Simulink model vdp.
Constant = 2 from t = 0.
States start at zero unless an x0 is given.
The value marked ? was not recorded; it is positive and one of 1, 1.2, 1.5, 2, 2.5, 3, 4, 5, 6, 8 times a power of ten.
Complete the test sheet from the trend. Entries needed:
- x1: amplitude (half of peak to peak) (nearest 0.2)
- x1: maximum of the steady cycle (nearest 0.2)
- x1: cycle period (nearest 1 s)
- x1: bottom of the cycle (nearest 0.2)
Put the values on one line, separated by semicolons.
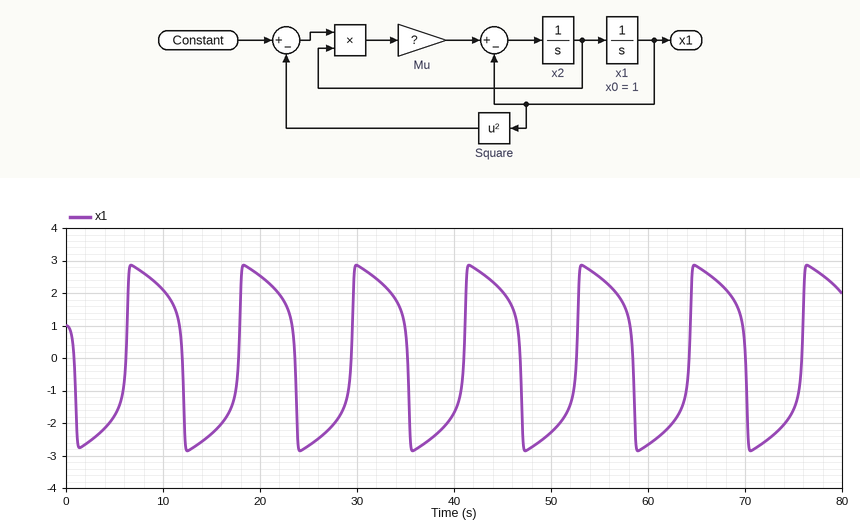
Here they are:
2.8; 2.8; 12 s; -2.8
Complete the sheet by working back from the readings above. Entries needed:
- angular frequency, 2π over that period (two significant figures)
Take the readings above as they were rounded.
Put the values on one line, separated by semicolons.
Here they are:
0.52 rad/s
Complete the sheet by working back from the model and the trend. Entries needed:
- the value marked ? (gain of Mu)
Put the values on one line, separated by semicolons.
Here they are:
2.5
